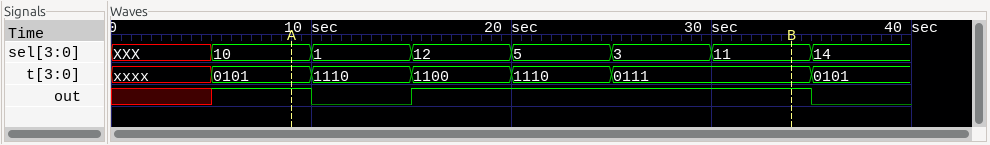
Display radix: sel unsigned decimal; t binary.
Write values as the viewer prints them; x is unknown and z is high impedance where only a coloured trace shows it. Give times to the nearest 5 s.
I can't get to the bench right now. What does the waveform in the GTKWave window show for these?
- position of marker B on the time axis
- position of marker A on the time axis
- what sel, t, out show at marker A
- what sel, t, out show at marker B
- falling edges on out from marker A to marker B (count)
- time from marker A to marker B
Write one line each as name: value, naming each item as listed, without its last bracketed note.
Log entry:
position of marker B on the time axis: 35 s
position of marker A on the time axis: 10 s
what sel, t, out show at marker A: sel=10, t=0101, out=1
what sel, t, out show at marker B: sel=11, t=0111, out=1
falling edges on out from marker A to marker B: 1
time from marker A to marker B: 25 s
